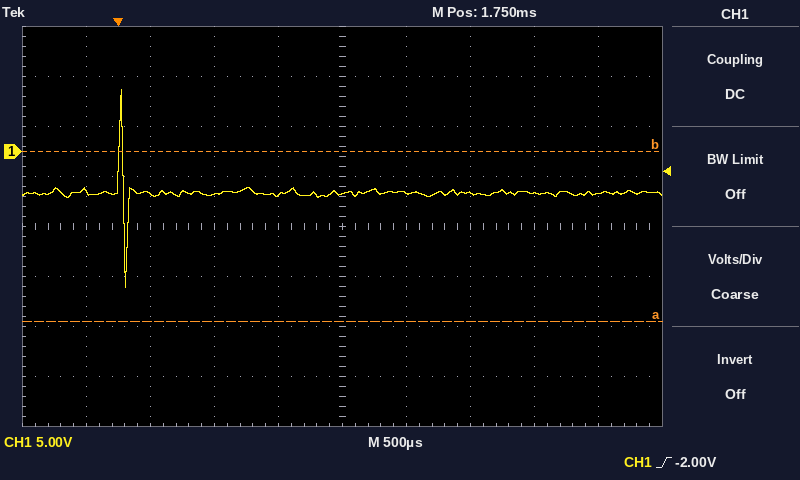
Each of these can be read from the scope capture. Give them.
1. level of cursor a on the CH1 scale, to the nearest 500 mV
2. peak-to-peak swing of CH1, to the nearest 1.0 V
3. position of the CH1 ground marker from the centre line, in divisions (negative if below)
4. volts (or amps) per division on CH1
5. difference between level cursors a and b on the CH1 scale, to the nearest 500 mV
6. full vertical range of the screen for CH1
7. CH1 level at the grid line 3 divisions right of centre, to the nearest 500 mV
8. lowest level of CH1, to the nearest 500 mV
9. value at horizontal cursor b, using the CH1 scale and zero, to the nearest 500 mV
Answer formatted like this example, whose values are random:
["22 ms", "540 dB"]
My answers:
["-17.0 V", "20.0 V", "+1.5 div", "5 V", "17.0 V", "40 V", "-4.0 V", "-13.5 V", "0.0 V"]
